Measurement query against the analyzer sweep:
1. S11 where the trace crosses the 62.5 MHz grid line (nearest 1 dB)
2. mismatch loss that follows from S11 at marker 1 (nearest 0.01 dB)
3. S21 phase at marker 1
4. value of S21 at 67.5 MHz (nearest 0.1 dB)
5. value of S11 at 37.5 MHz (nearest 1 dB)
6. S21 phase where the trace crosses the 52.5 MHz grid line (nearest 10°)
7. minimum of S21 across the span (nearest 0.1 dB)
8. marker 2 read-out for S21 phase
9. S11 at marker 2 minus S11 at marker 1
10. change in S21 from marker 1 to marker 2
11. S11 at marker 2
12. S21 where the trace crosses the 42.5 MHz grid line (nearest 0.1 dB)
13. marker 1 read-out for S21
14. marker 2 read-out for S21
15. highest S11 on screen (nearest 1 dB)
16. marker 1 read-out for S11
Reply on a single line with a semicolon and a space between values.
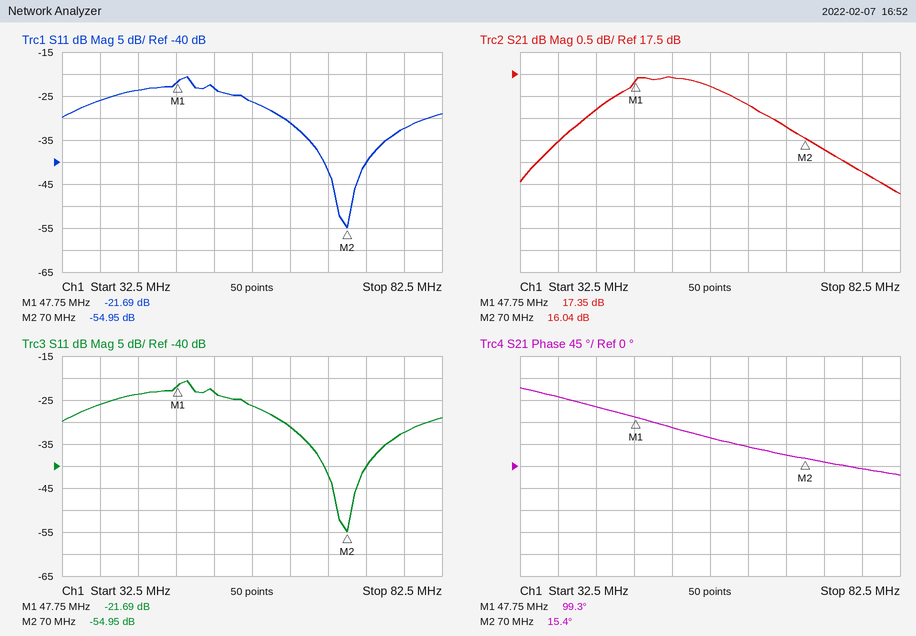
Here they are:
-31 dB; 0.03 dB; 99.3°; 16.3 dB; -26 dB; 80°; 14.8 dB; 15.4°; -33.26 dB; -1.31 dB; -54.95 dB; 16.7 dB; 17.35 dB; 16.04 dB; -21 dB; -21.69 dB
